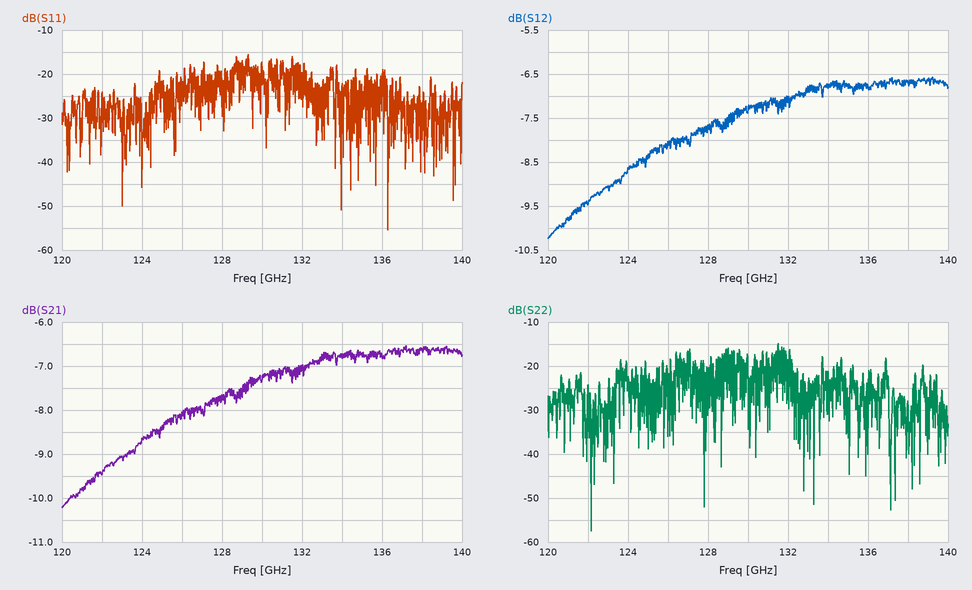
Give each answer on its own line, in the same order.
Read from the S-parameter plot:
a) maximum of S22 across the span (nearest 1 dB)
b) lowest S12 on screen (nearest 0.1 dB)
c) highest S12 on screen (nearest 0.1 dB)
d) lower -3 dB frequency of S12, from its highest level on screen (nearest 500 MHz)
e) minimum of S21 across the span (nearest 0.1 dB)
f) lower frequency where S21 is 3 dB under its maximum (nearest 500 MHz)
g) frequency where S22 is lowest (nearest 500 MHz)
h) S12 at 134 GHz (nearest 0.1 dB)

-15 dB
-10.2 dB
-6.6 dB
121.5 GHz
-10.2 dB
121.5 GHz
122.0 GHz
-6.8 dB
